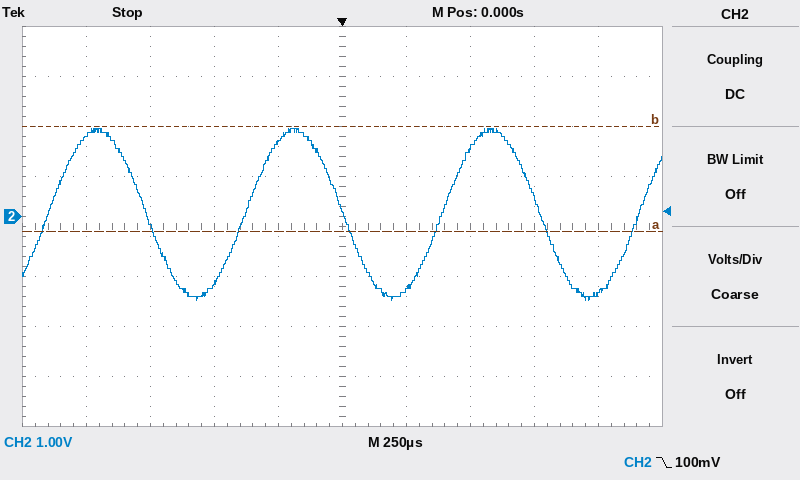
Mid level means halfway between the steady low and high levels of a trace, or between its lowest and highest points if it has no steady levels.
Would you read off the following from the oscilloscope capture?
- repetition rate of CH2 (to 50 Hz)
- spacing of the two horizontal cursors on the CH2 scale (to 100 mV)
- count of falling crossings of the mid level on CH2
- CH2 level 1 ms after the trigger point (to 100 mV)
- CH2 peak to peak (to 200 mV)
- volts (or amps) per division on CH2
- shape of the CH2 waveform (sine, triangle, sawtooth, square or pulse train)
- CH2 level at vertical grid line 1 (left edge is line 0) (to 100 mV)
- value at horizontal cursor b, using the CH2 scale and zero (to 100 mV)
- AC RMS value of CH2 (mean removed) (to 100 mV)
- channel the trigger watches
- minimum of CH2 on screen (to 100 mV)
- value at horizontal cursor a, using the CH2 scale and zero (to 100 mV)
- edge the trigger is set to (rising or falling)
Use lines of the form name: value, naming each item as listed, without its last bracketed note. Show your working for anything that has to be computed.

repetition rate of CH2: 1.30 kHz
spacing of the two horizontal cursors on the CH2 scale: 2.1 V
count of falling crossings of the mid level on CH2: 3
CH2 level 1 ms after the trigger point: -1.5 V
CH2 peak to peak: 3.4 V
volts (or amps) per division on CH2: 1 V
shape of the CH2 waveform: sine
CH2 level at vertical grid line 1 (left edge is line 0): 1.6 V
value at horizontal cursor b, using the CH2 scale and zero: 1.8 V
AC RMS value of CH2 (mean removed): 3.4 V / (2√2) ≈ 1.2 V
channel the trigger watches: CH2
minimum of CH2 on screen: -1.7 V
value at horizontal cursor a, using the CH2 scale and zero: -300 mV
edge the trigger is set to: falling
